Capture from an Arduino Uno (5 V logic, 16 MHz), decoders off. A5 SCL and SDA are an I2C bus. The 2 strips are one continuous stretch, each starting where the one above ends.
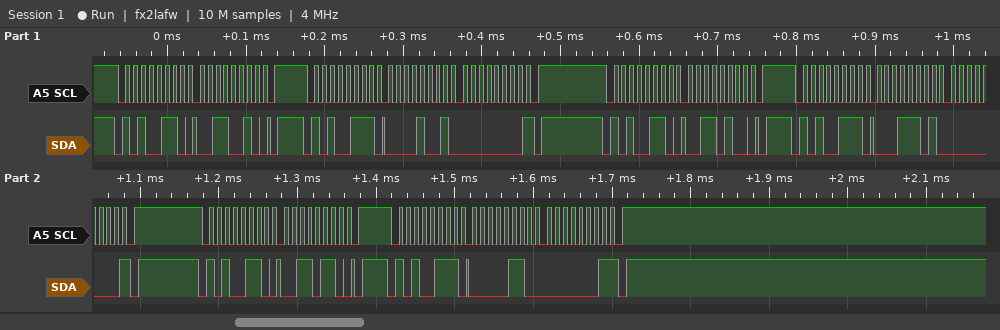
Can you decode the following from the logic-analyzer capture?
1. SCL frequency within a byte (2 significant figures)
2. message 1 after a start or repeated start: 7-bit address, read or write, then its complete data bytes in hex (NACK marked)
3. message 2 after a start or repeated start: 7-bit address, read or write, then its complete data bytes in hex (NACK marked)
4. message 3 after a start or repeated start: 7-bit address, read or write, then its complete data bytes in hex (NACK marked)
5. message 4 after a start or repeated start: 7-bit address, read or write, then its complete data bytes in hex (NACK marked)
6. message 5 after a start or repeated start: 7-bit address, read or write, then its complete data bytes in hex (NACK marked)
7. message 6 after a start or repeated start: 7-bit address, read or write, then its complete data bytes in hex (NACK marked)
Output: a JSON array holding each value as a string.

["100 kHz", "0x53 write: 32", "0x53 read: 09 00 NACK", "0x53 write: 34", "0x53 read: 1D 00 NACK", "0x53 write: 36", "0x53 read: 06 01 NACK"]
